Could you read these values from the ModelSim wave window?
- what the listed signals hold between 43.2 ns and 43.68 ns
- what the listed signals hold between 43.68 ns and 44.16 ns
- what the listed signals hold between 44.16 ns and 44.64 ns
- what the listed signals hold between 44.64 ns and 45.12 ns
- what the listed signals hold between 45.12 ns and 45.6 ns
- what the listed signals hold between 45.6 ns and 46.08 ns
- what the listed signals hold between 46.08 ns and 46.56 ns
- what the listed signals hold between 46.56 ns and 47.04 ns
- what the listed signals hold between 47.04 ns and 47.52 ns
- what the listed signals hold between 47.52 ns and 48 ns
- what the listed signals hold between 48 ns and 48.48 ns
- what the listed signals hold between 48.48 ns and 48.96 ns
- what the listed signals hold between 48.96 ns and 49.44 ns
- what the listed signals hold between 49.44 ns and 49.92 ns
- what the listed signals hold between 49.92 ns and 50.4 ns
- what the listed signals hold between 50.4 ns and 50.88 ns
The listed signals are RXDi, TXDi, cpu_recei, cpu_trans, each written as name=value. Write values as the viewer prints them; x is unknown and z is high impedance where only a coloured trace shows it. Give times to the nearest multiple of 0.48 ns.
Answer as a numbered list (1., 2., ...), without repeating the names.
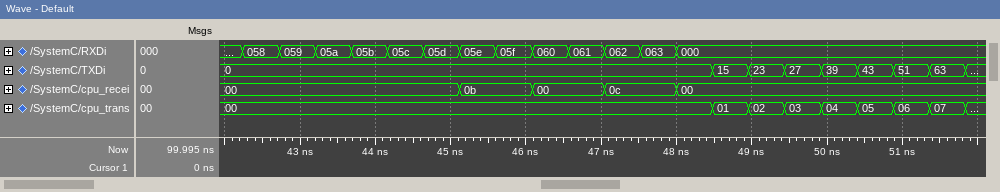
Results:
1. RXDi=05a, TXDi=0, cpu_recei=00, cpu_trans=00
2. RXDi=05b, TXDi=0, cpu_recei=00, cpu_trans=00
3. RXDi=05c, TXDi=0, cpu_recei=00, cpu_trans=00
4. RXDi=05d, TXDi=0, cpu_recei=00, cpu_trans=00
5. RXDi=05e, TXDi=0, cpu_recei=0b, cpu_trans=00
6. RXDi=05f, TXDi=0, cpu_recei=0b, cpu_trans=00
7. RXDi=060, TXDi=0, cpu_recei=00, cpu_trans=00
8. RXDi=061, TXDi=0, cpu_recei=00, cpu_trans=00
9. RXDi=062, TXDi=0, cpu_recei=0c, cpu_trans=00
10. RXDi=063, TXDi=0, cpu_recei=0c, cpu_trans=00
11. RXDi=000, TXDi=0, cpu_recei=00, cpu_trans=00
12. RXDi=000, TXDi=15, cpu_recei=00, cpu_trans=01
13. RXDi=000, TXDi=23, cpu_recei=00, cpu_trans=02
14. RXDi=000, TXDi=27, cpu_recei=00, cpu_trans=03
15. RXDi=000, TXDi=39, cpu_recei=00, cpu_trans=04
16. RXDi=000, TXDi=43, cpu_recei=00, cpu_trans=05
